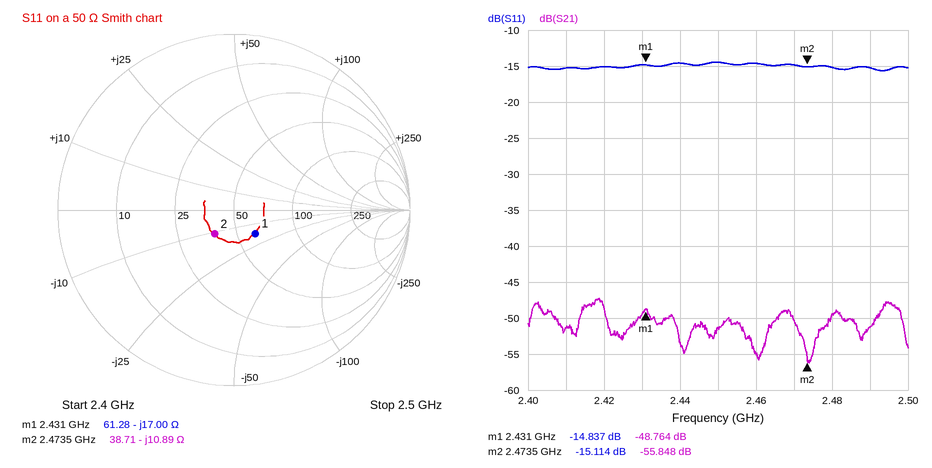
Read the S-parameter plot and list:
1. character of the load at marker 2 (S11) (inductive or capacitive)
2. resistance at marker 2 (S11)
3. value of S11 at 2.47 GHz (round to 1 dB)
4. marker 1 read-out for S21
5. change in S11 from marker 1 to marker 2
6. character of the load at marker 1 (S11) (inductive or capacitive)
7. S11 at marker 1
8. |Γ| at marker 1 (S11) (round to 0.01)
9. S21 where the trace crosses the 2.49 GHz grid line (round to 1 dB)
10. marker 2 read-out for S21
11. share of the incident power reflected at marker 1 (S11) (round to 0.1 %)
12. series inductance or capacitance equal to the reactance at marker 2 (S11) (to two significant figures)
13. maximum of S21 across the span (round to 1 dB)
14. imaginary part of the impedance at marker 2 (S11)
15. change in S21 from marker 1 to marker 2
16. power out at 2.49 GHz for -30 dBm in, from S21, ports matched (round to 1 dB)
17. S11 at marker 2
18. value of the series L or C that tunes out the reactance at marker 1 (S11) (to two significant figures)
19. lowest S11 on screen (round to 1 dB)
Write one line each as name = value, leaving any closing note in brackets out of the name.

character of the load at marker 2 (S11) = capacitive
resistance at marker 2 = 38.71 Ω
value of S11 at 2.47 GHz = -15 dB
marker 1 read-out for S21 = -48.764 dB
change in S11 from marker 1 to marker 2 = -0.277 dB
character of the load at marker 1 (S11) = capacitive
S11 at marker 1 = -14.837 dB
|Γ| at marker 1 (S11) = 0.18
S21 where the trace crosses the 2.49 GHz grid line = -51 dB
marker 2 read-out for S21 = -55.848 dB
share of the incident power reflected at marker 1 (S11) = 3.3 %
series inductance or capacitance equal to the reactance at marker 2 (S11) = 5.9 pF
maximum of S21 across the span = -47 dB
imaginary part of the impedance at marker 2 = -10.89 Ω
change in S21 from marker 1 to marker 2 = -7.084 dB
power out at 2.49 GHz for -30 dBm in, from S21, ports matched = -81 dBm
S11 at marker 2 = -15.114 dB
value of the series L or C that tunes out the reactance at marker 1 (S11) = 1.1 nH
lowest S11 on screen = -16 dB
